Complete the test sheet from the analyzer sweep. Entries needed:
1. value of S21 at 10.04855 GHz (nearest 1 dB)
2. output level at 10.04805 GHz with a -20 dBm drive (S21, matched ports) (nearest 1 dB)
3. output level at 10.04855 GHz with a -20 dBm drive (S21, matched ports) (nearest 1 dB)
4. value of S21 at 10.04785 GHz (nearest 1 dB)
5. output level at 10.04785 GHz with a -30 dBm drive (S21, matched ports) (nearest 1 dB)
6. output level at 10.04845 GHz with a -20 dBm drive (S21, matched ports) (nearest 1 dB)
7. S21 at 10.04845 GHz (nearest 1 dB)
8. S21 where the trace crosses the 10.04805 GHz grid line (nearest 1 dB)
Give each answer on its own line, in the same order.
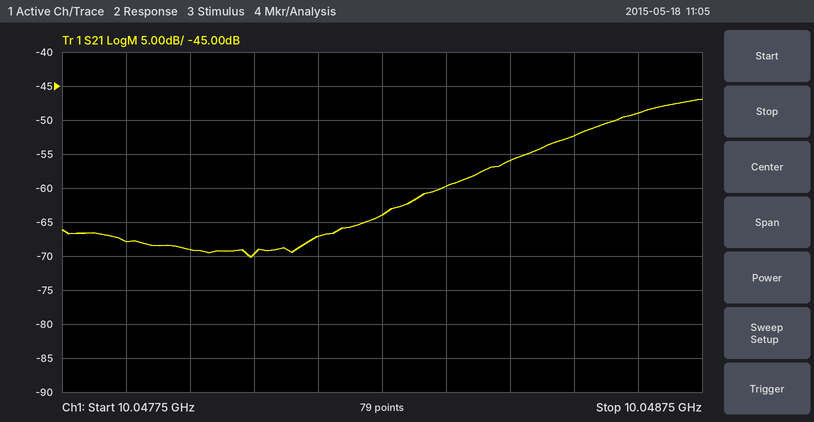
-52 dB
-90 dBm
-72 dBm
-68 dB
-98 dBm
-76 dBm
-56 dB
-70 dB
